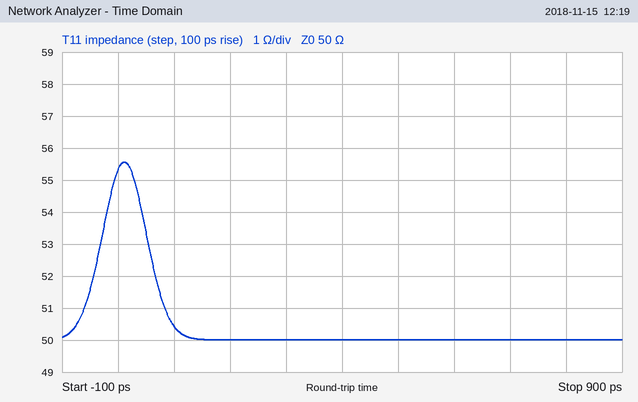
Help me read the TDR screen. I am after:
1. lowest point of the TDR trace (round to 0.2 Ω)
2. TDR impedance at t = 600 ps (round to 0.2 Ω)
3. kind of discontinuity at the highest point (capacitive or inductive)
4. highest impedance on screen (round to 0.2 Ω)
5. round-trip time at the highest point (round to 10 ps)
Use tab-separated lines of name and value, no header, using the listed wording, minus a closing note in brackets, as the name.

lowest point of the TDR trace	50.0 Ω
TDR impedance at t = 600 ps	50.0 Ω
kind of discontinuity at the highest point	inductive
highest impedance on screen	55.6 Ω
round-trip time at the highest point	10 ps
